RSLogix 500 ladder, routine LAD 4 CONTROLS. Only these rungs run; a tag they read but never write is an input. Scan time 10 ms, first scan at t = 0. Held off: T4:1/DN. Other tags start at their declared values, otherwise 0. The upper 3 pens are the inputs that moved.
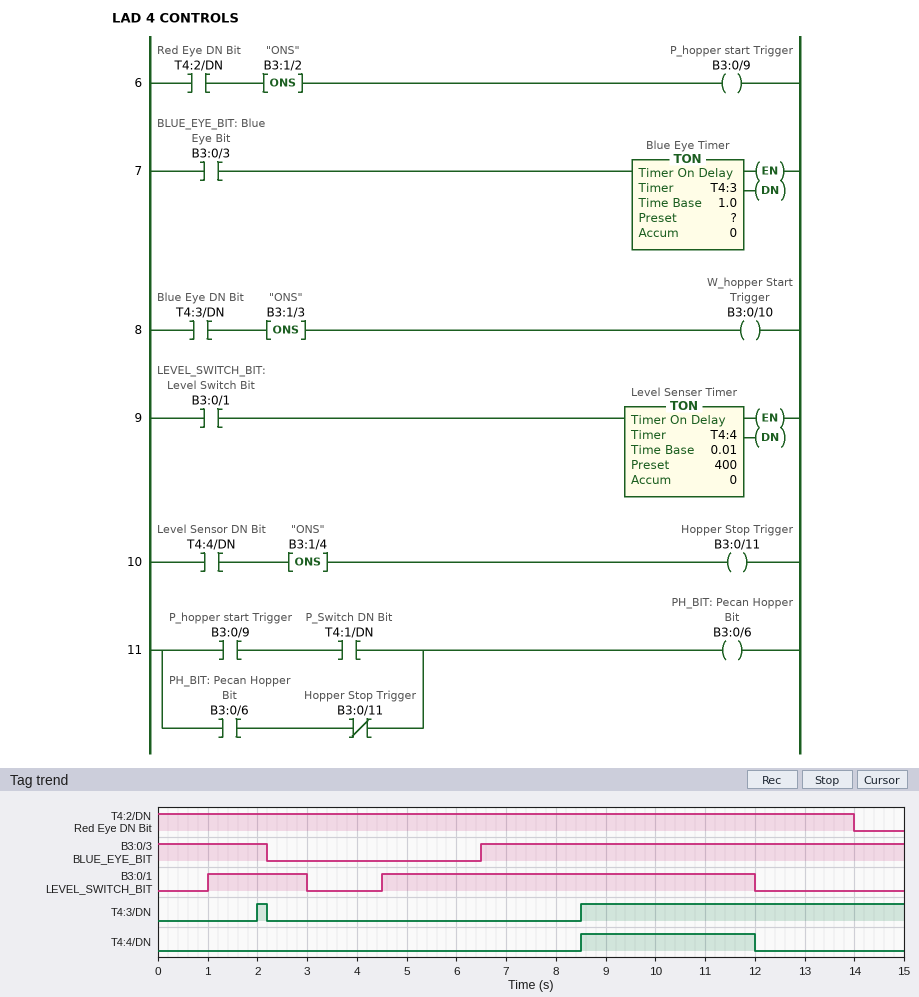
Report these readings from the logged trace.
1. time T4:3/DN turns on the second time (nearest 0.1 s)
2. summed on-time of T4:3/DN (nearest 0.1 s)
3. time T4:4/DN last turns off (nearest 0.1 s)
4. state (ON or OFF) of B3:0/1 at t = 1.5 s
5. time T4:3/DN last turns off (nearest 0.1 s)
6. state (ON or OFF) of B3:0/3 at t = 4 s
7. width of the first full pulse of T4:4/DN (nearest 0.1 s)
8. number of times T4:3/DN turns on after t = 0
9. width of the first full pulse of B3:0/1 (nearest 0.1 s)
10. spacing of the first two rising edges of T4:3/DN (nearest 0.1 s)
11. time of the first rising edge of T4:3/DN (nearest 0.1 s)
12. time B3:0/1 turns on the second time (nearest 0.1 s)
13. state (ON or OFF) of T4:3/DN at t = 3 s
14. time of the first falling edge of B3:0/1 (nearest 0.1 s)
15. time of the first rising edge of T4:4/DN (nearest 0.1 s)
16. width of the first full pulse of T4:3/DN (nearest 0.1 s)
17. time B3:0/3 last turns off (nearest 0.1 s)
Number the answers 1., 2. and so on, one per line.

1. 8.5 s
2. 6.7 s
3. 12.0 s
4. ON
5. 2.2 s
6. OFF
7. 3.5 s
8. 2
9. 2.0 s
10. 6.5 s
11. 2.0 s
12. 4.5 s
13. OFF
14. 3.0 s
15. 8.5 s
16. 0.2 s
17. 2.2 s
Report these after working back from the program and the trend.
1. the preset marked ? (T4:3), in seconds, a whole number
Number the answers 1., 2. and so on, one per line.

1. 2 s
